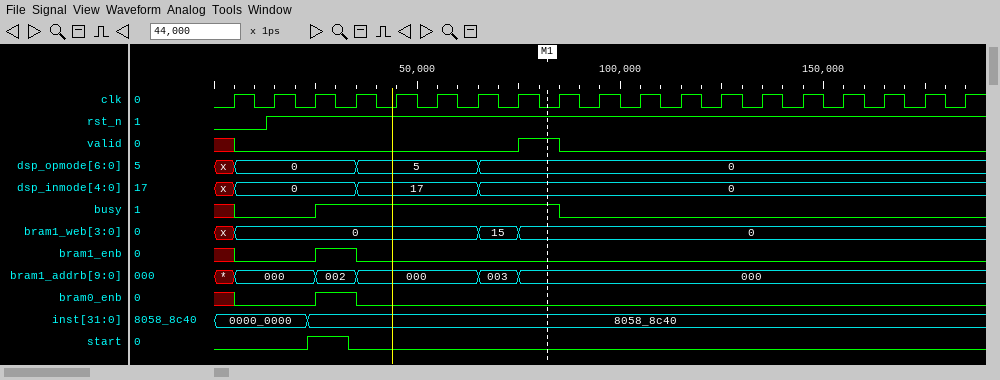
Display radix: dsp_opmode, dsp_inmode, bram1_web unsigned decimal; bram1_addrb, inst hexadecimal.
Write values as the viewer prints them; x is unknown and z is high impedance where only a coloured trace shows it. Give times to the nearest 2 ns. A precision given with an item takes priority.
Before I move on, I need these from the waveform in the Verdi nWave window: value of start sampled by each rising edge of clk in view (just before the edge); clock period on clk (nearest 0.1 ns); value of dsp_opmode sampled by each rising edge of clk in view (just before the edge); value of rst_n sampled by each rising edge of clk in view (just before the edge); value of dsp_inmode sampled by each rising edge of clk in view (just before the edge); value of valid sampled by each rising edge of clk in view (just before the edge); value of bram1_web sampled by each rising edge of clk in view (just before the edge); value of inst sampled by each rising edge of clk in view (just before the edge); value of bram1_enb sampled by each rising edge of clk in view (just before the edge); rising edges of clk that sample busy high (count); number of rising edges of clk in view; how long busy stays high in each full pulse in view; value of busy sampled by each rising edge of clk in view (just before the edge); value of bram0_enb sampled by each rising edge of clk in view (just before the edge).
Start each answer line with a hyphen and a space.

- 0 0 1 0 0 0 0 0 0 0 0 0 0 0 0 0 0 0 0
- 10 ns
- x, 0, 0, 0, 5, 5, 5, 0, 0, 0, 0, 0, 0, 0, 0, 0, 0, 0, 0
- 0 1 1 1 1 1 1 1 1 1 1 1 1 1 1 1 1 1 1
- x, 0, 0, 0, 17, 17, 17, 0, 0, 0, 0, 0, 0, 0, 0, 0, 0, 0, 0
- x 0 0 0 0 0 0 0 1 0 0 0 0 0 0 0 0 0 0
- x, 0, 0, 0, 0, 0, 0, 15, 0, 0, 0, 0, 0, 0, 0, 0, 0, 0, 0
- 0000_0000, 0000_0000, 8058_8c40, 8058_8c40, 8058_8c40, 8058_8c40, 8058_8c40, 8058_8c40, 8058_8c40, 8058_8c40, 8058_8c40, 8058_8c40, 8058_8c40, 8058_8c40, 8058_8c40, 8058_8c40, 8058_8c40, 8058_8c40, 8058_8c40
- x 0 0 1 0 0 0 0 0 0 0 0 0 0 0 0 0 0 0
- 6
- 19
- 60 ns
- x 0 0 1 1 1 1 1 1 0 0 0 0 0 0 0 0 0 0
- x 0 0 1 0 0 0 0 0 0 0 0 0 0 0 0 0 0 0
